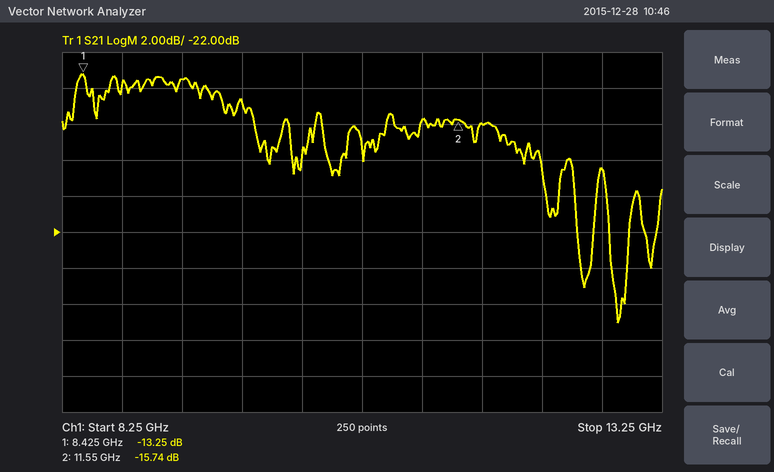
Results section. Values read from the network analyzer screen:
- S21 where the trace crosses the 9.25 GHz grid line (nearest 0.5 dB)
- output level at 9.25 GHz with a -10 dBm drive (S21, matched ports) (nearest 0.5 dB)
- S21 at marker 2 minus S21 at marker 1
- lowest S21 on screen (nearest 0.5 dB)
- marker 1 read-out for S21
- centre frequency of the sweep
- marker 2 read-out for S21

-13.5 dB
-23.5 dBm
-2.49 dB
-27.0 dB
-13.25 dB
10.75 GHz
-15.74 dB
